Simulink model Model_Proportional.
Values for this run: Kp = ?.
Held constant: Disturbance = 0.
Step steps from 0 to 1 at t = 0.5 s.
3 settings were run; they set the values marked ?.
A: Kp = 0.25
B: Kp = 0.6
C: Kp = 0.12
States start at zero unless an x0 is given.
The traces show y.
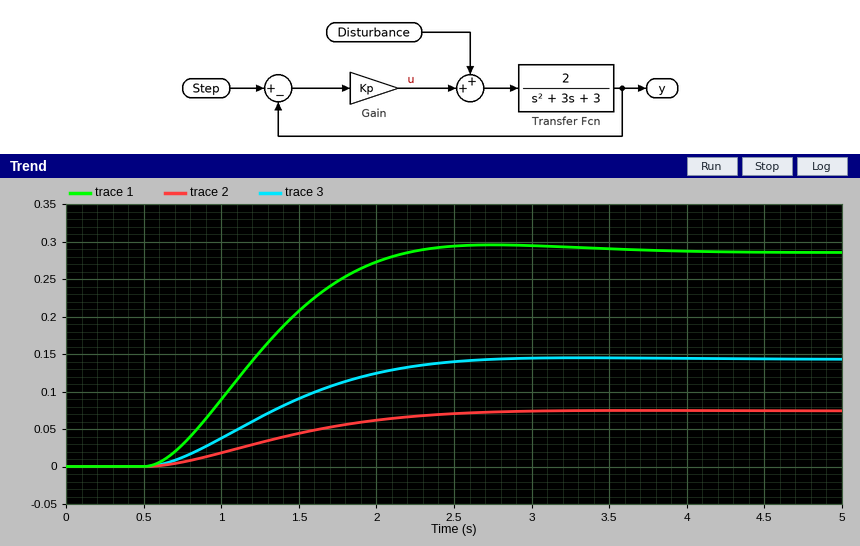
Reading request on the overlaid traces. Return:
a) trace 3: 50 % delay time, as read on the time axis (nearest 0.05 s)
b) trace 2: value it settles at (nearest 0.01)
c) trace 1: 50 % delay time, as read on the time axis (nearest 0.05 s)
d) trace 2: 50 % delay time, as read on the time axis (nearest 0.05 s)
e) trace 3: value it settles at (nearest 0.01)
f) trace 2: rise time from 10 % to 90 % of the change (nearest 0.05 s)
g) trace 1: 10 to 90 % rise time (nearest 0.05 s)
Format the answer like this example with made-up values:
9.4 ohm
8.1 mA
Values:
1.30 s
0.07
1.20 s
1.35 s
0.14
1.45 s
1.10 s
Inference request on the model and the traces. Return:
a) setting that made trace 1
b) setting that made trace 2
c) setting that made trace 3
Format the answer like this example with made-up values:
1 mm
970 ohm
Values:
B
C
A
